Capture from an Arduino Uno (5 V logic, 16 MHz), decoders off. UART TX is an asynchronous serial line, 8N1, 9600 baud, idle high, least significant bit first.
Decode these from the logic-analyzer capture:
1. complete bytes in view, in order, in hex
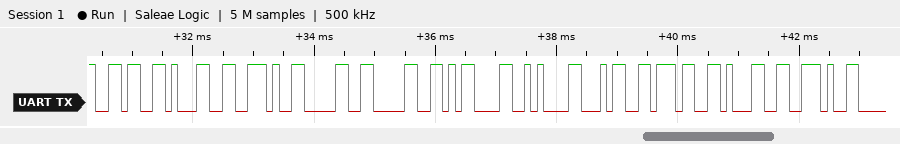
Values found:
0x36 0x31 0x2E 0x30 0x30 0x0D 0x0A 0x34 0x37 0x31 0x2E
